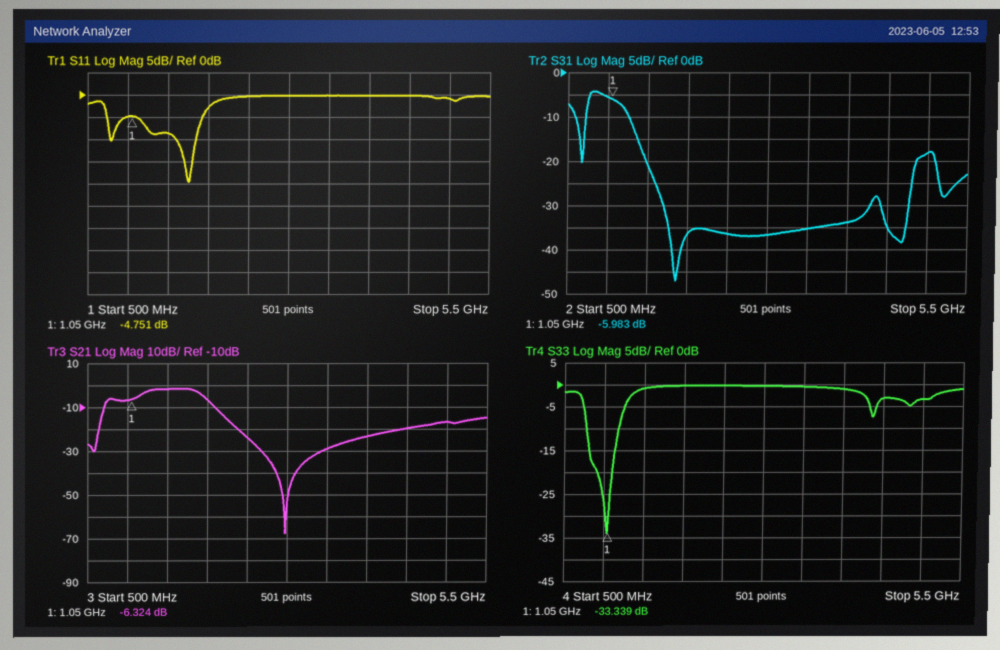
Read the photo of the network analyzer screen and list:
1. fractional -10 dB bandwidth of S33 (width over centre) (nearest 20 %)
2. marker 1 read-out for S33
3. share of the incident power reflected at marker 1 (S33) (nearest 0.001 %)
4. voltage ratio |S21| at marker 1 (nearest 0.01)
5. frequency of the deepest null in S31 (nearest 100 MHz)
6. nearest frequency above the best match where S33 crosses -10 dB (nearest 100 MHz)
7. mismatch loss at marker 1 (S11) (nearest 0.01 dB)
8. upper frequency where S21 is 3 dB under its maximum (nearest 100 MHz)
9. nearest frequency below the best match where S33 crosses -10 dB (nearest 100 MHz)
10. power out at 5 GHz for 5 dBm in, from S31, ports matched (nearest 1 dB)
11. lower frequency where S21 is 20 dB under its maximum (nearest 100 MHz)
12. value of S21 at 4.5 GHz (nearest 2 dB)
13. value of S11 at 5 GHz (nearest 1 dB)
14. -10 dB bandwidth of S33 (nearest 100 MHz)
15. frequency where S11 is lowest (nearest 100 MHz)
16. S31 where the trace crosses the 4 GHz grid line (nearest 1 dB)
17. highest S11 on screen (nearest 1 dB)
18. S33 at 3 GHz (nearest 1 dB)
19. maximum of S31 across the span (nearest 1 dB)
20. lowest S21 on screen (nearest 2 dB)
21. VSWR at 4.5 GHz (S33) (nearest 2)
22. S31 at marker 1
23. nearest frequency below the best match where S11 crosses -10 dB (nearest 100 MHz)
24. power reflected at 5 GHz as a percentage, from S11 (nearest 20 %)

40 %
-33.339 dB
0.046 %
0.48
1.9 GHz
1.2 GHz
1.77 dB
1.9 GHz
800 MHz
-13 dBm
600 MHz
-20 dB
-1 dB
400 MHz
1.8 GHz
-34 dB
0 dB
0 dB
-4 dB
-68 dB
6
-5.983 dB
1.6 GHz
80 %
